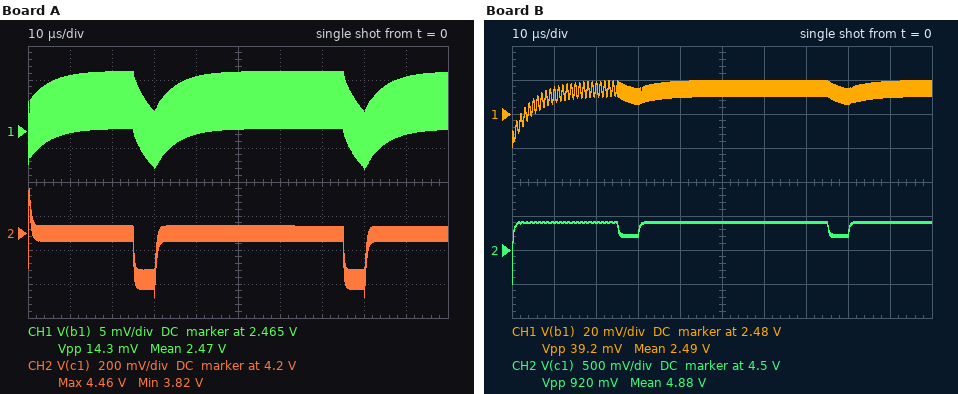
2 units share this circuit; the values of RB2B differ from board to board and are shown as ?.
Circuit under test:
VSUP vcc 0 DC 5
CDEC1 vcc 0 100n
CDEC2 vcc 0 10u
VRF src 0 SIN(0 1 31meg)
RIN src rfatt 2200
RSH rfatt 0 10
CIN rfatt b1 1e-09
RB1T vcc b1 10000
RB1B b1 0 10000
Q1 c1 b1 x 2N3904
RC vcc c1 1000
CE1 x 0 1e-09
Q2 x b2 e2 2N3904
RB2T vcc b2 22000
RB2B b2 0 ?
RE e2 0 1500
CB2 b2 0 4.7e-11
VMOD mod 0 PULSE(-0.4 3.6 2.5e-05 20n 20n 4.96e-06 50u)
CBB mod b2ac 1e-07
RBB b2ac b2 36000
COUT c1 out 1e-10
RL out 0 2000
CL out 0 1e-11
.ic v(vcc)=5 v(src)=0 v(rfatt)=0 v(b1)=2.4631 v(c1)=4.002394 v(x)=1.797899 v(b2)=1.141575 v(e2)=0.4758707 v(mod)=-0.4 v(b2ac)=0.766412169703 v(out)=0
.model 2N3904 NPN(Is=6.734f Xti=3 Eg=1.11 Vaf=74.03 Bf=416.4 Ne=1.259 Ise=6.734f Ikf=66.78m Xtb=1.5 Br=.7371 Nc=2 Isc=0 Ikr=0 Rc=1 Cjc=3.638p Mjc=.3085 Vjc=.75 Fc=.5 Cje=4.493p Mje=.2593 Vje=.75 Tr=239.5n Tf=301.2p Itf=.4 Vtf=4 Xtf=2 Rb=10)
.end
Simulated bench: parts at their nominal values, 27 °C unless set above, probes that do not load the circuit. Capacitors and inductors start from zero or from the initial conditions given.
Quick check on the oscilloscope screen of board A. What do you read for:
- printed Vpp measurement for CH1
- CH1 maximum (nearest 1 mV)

14.3 mV
2.474 V
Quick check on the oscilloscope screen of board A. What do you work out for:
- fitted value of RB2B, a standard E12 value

18 kΩ
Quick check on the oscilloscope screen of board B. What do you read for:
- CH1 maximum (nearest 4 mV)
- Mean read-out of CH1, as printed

2.500 V
2.49 V
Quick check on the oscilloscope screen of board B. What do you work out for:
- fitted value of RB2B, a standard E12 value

3.9 kΩ
